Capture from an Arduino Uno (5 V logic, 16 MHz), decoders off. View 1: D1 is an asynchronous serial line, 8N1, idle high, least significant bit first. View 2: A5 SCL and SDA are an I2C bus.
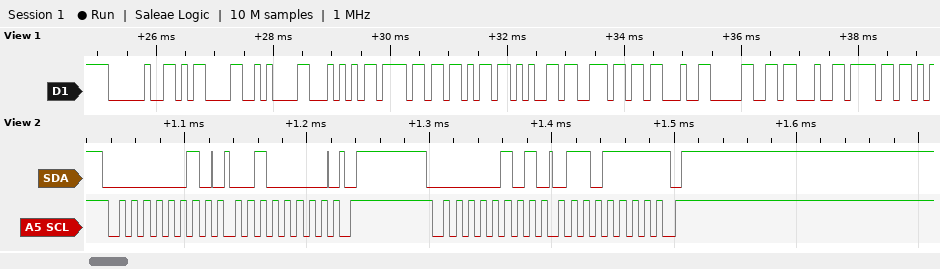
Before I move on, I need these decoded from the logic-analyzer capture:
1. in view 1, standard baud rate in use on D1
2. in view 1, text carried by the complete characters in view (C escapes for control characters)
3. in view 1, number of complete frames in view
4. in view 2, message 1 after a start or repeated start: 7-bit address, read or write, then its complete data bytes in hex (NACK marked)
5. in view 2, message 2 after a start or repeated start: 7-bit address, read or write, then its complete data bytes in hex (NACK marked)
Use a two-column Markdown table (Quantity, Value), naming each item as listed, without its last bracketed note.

| Quantity | Value |
|---|---|
| in view 1, standard baud rate in use on D1 | 9600 baud |
| in view 1, text carried by the complete characters in view | " \r\nToken#0#o" |
| in view 1, number of complete frames in view | 12 |
| in view 2, message 1 after a start or repeated start: 7-bit address, read or write, then its complete data bytes in hex | 0x01 write: 20 |
| in view 2, message 2 after a start or repeated start: 7-bit address, read or write, then its complete data bytes in hex | 0x02 read: 6F NACK |
